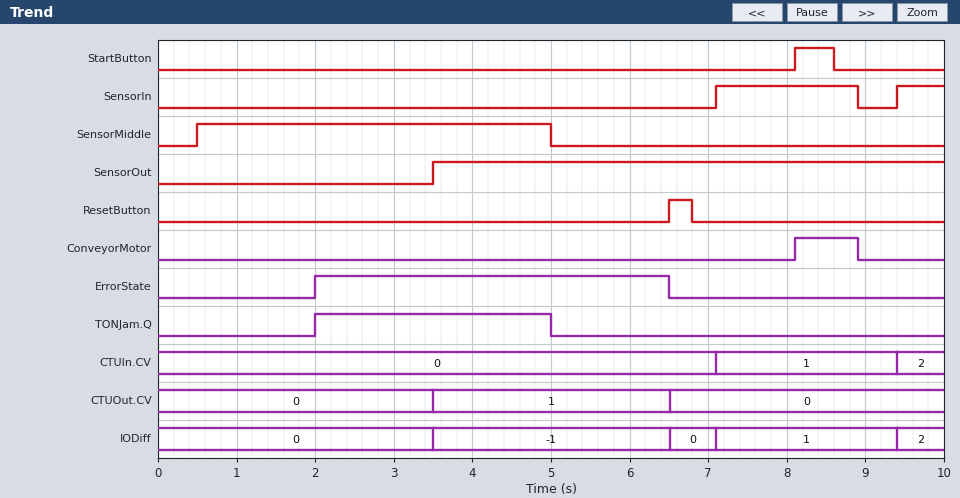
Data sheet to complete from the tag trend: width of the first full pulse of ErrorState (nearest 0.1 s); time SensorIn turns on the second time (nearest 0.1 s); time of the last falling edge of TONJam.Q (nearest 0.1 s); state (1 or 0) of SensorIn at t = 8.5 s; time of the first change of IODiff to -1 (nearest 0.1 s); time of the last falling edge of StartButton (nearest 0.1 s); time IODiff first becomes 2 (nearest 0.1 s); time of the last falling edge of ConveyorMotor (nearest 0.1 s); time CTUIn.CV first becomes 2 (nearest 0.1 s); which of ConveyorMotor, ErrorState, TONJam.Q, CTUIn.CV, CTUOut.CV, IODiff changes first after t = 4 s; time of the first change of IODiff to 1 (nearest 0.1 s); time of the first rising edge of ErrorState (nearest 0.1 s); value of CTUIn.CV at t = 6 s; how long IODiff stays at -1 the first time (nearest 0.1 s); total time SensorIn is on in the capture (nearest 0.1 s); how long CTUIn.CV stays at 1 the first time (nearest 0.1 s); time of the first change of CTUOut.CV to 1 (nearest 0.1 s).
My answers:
4.5 s
9.4 s
5.0 s
1
3.5 s
8.6 s
9.4 s
8.9 s
9.4 s
TONJam.Q
7.1 s
2.0 s
0
3.0 s
2.4 s
2.3 s
3.5 s
